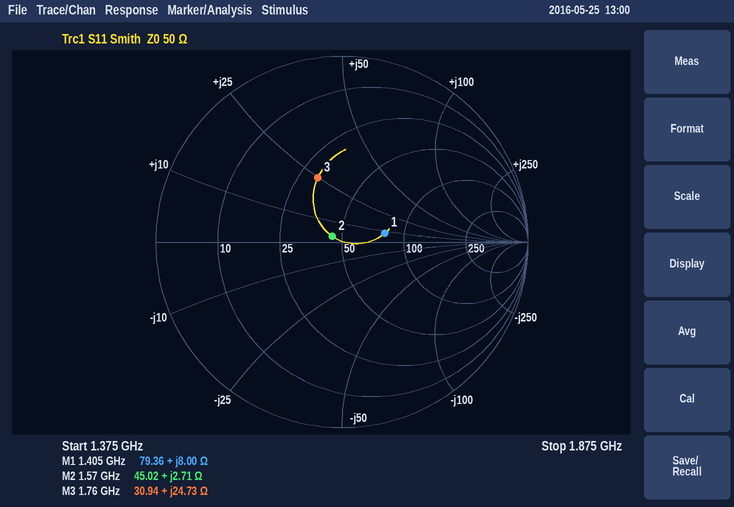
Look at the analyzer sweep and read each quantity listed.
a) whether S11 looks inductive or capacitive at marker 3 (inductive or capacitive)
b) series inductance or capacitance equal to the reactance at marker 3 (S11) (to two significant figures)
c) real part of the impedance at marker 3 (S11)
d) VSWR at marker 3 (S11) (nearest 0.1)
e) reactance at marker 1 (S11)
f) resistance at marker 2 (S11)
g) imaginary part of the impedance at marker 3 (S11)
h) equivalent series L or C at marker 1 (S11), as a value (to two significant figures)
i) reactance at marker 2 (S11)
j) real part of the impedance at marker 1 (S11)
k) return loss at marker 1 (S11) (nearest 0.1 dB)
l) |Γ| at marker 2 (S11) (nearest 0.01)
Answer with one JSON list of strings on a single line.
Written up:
["inductive", "2.2 nH", "30.94 Ω", "2.2", "+8.00 Ω", "45.02 Ω", "+24.73 Ω", "910 pH", "+2.71 Ω", "79.36 Ω", "12.6 dB", "0.06"]
